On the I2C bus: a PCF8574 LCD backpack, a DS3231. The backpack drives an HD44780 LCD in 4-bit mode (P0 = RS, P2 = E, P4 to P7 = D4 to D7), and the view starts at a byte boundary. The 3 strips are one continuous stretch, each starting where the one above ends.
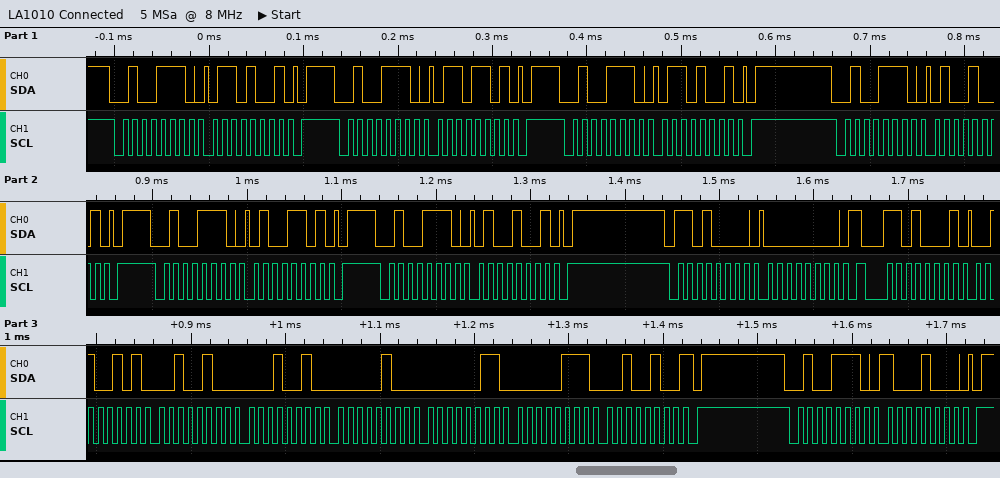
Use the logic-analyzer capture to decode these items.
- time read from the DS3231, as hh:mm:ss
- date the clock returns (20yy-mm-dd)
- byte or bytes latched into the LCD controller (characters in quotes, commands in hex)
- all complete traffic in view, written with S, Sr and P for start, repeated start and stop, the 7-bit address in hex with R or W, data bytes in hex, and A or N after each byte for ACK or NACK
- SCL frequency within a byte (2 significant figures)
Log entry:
12:24:25
2024-07-03
'd'
S 27W A 69 A P S 27W A 6D A P S 27W A 69 A P S 27W A 49 A P S 27W A 4D A P S 27W A 49 A P S 68W A 00 A Sr 68R A 25 A 24 A 12 A 04 A 03 A 07 A 24 N P S 27W A 88 A P
100 kHz
